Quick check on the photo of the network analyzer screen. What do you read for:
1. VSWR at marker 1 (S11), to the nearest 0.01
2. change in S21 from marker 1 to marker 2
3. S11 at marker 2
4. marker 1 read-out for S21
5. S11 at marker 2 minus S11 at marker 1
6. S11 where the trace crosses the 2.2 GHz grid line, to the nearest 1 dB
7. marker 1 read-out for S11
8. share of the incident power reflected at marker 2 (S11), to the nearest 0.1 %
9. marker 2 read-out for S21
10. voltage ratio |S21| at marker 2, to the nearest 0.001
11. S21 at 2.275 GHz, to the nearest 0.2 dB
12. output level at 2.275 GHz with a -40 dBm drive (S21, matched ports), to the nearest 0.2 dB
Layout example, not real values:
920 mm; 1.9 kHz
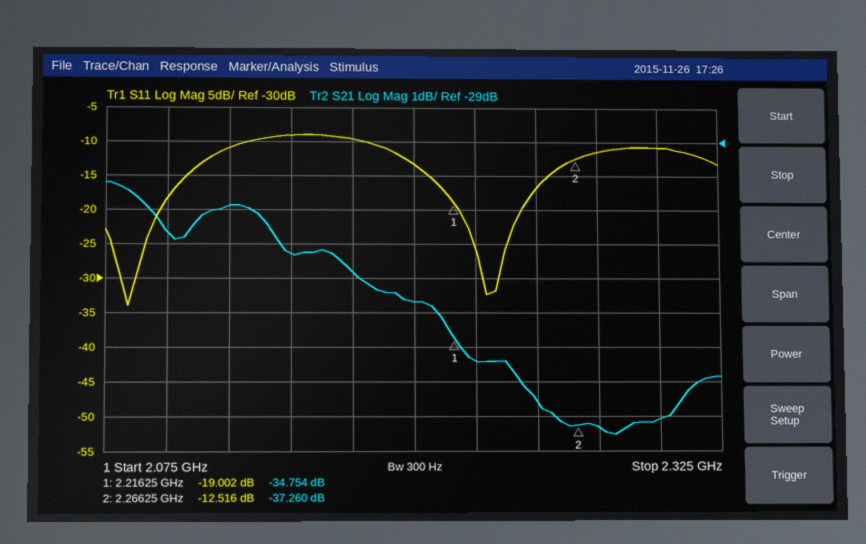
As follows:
1.25; -2.506 dB; -12.516 dB; -34.754 dB; 6.486 dB; -13 dB; -19.002 dB; 5.6 %; -37.260 dB; 0.014; -37.4 dB; -77.4 dBm
